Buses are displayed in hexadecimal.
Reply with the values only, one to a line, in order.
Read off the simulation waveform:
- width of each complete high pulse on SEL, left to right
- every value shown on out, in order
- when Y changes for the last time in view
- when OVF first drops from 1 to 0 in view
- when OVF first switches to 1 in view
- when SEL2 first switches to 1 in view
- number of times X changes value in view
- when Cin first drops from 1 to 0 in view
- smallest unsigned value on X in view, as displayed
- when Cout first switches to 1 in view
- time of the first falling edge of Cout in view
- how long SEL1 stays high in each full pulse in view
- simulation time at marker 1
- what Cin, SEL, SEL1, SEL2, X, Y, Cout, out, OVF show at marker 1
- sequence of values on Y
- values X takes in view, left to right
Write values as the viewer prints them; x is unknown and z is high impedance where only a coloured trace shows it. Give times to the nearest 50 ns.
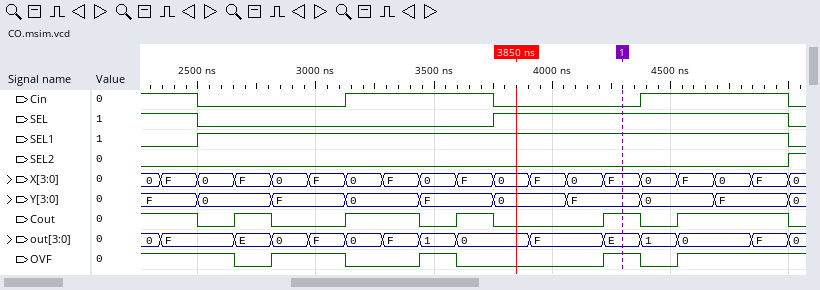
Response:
1250 ns
0, F, E, 0, F, 0, F, 1, 0, F, E, 1, 0, F, 0
5000 ns
2650 ns
2800 ns
5000 ns
18
2500 ns
0
2650 ns
2500 ns
2500 ns
4300 ns
Cin=0, SEL=1, SEL1=1, SEL2=0, X=F, Y=F, Cout=1, out=E, OVF=1
F, 0, F, 0, F, 0, F, 0, F, 0
0, F, 0, F, 0, F, 0, F, 0, F, 0, F, 0, F, 0, F, 0, F, 0
